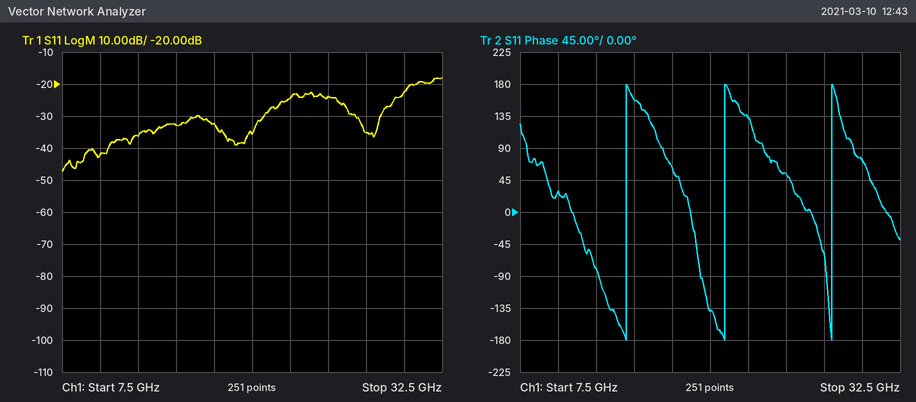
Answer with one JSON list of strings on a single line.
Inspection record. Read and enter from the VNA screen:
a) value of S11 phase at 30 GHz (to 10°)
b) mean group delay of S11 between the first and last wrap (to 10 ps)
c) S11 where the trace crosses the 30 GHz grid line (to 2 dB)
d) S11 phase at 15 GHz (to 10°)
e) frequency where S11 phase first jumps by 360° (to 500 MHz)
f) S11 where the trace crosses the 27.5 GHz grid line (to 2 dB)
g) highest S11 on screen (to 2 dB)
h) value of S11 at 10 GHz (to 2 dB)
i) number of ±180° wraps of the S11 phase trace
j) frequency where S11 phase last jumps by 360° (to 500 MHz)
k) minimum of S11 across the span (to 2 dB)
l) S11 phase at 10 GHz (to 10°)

["70°", "150 ps", "-22 dB", "160°", "14.5 GHz", "-36 dB", "-18 dB", "-42 dB", "3", "28.0 GHz", "-48 dB", "30°"]
